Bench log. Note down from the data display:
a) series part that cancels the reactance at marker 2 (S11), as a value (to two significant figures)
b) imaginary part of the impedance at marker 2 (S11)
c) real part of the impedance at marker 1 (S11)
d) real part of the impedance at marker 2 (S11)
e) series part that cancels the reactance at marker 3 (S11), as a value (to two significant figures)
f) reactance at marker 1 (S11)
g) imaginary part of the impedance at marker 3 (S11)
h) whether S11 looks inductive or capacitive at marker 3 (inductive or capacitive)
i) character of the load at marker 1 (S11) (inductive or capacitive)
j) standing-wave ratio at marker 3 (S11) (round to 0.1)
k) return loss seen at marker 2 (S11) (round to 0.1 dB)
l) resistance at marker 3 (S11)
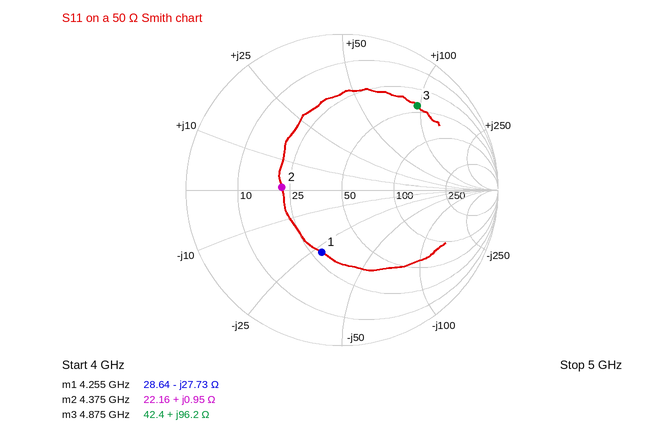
38 pF
+0.95 Ω
28.64 Ω
22.16 Ω
340 fF
-27.73 Ω
+96.2 Ω
inductive
capacitive
6.2
8.3 dB
42.4 Ω
